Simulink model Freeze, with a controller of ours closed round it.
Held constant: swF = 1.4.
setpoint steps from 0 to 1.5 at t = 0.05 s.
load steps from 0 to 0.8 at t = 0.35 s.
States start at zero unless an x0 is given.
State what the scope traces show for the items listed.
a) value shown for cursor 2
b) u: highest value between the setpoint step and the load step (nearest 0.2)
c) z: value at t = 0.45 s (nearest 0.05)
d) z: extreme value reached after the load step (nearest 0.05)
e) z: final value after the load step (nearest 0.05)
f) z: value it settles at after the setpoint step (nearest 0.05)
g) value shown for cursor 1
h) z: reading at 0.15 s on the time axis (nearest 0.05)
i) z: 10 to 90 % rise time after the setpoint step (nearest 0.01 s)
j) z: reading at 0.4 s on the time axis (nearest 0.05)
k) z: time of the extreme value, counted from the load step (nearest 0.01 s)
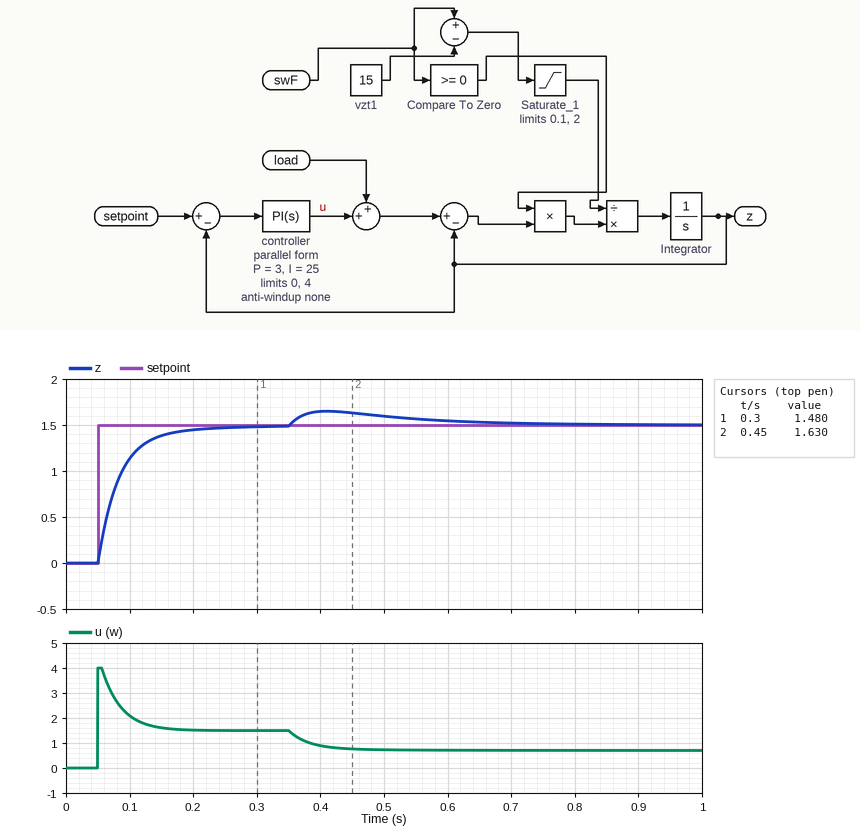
1.630
4.0
1.65
1.65
1.50
1.50
1.480
1.40
0.08 s
1.65
0.06 s
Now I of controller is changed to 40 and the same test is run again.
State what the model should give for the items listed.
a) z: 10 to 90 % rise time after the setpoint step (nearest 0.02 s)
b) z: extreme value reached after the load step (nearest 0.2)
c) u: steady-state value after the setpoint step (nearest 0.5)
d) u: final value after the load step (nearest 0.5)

0.06 s
1.6
1.5
0.5
